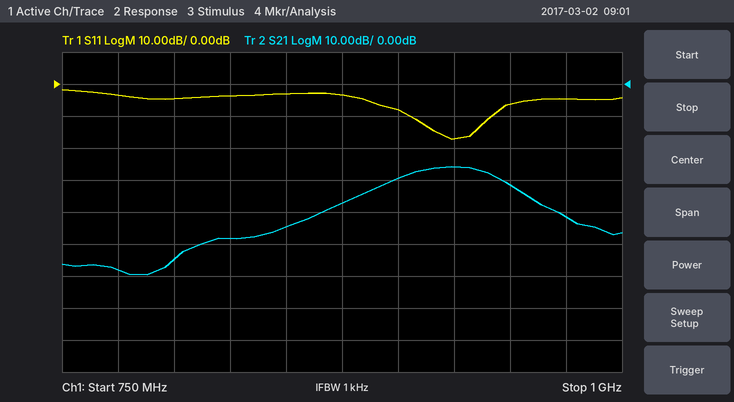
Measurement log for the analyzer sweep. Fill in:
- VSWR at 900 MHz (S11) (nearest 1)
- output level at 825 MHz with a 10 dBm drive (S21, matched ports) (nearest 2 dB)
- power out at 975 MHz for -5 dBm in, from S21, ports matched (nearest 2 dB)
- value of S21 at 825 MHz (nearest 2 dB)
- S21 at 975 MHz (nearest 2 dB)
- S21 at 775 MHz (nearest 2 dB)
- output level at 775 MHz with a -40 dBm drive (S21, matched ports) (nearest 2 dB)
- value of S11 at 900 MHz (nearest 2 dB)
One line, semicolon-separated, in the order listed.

2; -38 dBm; -46 dBm; -48 dB; -42 dB; -58 dB; -98 dBm; -8 dB
